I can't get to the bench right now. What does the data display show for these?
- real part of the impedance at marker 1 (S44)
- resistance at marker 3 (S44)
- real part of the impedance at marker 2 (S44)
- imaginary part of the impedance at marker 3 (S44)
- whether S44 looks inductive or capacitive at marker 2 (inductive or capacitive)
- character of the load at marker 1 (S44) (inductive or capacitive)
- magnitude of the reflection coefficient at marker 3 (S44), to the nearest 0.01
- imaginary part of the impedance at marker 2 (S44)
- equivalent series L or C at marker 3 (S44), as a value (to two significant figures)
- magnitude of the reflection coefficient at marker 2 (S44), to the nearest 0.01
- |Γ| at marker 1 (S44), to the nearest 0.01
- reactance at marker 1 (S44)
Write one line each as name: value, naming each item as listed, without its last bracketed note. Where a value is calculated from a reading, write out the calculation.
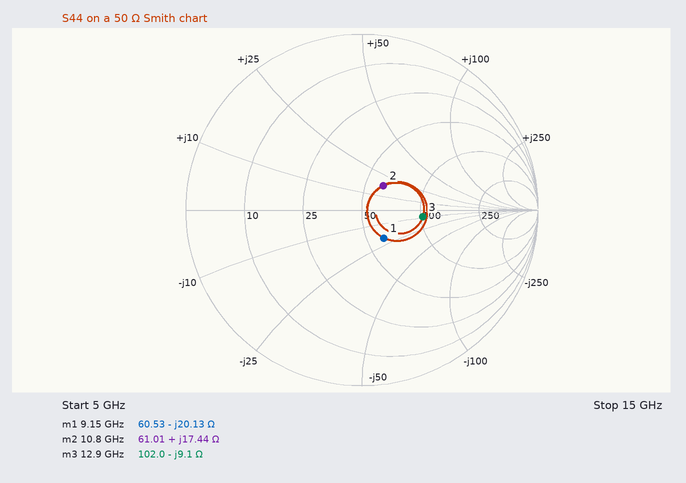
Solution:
real part of the impedance at marker 1: 60.53 Ω
resistance at marker 3: 102.0 Ω
real part of the impedance at marker 2: 61.01 Ω
imaginary part of the impedance at marker 3: -9.1 Ω
whether S44 looks inductive or capacitive at marker 2: inductive
character of the load at marker 1 (S44): capacitive
magnitude of the reflection coefficient at marker 3 (S44), to the nearest 0.01: 0.35
imaginary part of the impedance at marker 2: +17.44 Ω
equivalent series L or C at marker 3 (S44), as a value: C = 1/(2π × 12.9 GHz × 9.1 Ω) ≈ 1.4 pF
magnitude of the reflection coefficient at marker 2 (S44), to the nearest 0.01: 0.18
|Γ| at marker 1 (S44), to the nearest 0.01: 0.20
reactance at marker 1: -20.13 Ω
